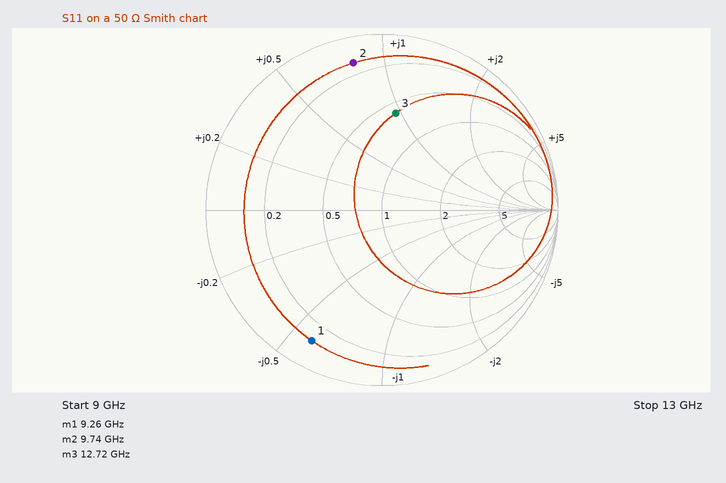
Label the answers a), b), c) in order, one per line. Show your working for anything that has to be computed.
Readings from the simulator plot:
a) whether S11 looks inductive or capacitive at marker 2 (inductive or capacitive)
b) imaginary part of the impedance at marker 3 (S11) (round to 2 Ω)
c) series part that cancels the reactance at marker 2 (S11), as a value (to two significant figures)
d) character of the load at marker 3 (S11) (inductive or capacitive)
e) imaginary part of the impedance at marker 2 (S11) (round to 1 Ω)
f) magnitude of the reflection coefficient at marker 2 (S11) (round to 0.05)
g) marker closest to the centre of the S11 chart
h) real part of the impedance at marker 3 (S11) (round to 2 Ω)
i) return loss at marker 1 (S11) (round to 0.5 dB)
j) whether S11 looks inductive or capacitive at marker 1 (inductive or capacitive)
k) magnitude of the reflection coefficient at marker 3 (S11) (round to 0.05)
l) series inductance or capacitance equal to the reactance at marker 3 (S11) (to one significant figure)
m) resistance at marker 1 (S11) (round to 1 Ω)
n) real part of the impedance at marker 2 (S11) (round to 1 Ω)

a) inductive
b) +48 Ω
c) C = 1/(2π × 9.74 GHz × 41 Ω) ≈ 399 fF, so 400 fF to two significant figures
d) inductive
e) +41 Ω
f) 0.85
g) marker 3
h) 30 Ω
i) 1.5 dB
j) capacitive
k) 0.55
l) L = 48 Ω/(2π × 12.72 GHz) ≈ 601 pH, so 600 pH to one significant figure
m) 6 Ω
n) 7 Ω
